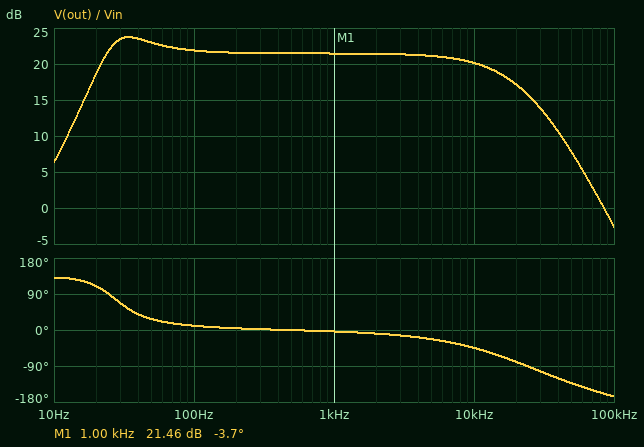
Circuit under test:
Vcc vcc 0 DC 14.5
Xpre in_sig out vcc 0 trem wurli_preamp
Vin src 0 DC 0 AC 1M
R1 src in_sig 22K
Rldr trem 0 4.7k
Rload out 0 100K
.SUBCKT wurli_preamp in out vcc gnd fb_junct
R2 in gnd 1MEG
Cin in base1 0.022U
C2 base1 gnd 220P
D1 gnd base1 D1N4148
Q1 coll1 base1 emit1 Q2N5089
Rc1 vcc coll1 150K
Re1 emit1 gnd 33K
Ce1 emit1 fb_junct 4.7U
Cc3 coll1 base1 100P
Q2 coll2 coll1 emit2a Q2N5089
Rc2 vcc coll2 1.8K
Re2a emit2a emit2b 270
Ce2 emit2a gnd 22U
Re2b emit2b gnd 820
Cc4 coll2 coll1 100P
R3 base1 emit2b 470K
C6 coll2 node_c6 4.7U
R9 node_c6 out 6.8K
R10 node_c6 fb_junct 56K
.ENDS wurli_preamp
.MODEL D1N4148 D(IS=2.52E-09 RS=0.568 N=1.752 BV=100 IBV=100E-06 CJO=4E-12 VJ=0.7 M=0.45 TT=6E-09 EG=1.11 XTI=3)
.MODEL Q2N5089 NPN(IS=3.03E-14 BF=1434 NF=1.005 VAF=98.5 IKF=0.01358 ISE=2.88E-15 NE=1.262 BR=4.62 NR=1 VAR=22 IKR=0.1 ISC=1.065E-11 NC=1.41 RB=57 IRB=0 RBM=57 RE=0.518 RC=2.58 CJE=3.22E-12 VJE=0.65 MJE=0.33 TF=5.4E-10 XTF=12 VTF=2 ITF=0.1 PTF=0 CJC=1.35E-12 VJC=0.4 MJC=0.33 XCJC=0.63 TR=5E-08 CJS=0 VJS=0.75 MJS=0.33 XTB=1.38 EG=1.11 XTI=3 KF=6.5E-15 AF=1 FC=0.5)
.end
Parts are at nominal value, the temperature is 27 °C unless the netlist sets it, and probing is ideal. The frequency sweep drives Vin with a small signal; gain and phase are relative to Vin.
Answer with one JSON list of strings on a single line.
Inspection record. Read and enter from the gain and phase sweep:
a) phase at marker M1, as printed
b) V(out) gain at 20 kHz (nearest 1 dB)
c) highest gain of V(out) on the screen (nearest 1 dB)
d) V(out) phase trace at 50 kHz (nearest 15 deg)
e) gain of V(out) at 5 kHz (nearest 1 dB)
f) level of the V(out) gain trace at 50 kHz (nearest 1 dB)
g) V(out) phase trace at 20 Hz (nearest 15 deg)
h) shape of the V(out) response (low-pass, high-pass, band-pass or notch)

["-3.7 deg", "17 dB", "24 dB", "-135 deg", "21 dB", "8 dB", "105 deg", "band-pass"]
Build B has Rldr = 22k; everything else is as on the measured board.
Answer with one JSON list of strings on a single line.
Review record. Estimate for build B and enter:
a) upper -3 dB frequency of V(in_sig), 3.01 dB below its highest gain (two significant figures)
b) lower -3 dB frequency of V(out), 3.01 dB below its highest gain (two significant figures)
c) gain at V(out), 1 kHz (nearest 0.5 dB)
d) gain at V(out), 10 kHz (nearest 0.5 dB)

["22 kHz", "16 Hz", "12.5 dB", "11.5 dB"]
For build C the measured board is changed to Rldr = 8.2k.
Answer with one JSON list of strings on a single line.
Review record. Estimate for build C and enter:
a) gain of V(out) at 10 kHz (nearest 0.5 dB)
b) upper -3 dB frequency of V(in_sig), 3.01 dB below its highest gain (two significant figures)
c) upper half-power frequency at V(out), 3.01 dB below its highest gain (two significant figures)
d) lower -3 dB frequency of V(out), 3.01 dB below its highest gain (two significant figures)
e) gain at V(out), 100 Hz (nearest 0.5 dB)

["16.5 dB", "22 kHz", "12 kHz", "19 Hz", "18.0 dB"]
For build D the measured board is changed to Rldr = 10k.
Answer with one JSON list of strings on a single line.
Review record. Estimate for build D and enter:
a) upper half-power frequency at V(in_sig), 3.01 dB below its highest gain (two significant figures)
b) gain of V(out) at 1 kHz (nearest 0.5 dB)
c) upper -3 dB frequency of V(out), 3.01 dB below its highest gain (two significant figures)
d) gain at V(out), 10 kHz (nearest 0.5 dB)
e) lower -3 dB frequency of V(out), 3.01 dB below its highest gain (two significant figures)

["22 kHz", "16.5 dB", "13 kHz", "15.5 dB", "18 Hz"]
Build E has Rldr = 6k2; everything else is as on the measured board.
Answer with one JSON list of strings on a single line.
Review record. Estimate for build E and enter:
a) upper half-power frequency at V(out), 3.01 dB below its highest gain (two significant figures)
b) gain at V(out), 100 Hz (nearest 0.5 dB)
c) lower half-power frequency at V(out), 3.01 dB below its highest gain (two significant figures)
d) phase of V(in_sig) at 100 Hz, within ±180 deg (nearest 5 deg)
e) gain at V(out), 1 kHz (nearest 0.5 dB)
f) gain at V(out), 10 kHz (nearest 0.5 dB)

["9.7 kHz", "20.0 dB", "21 Hz", "0 deg", "19.5 dB", "18.5 dB"]
